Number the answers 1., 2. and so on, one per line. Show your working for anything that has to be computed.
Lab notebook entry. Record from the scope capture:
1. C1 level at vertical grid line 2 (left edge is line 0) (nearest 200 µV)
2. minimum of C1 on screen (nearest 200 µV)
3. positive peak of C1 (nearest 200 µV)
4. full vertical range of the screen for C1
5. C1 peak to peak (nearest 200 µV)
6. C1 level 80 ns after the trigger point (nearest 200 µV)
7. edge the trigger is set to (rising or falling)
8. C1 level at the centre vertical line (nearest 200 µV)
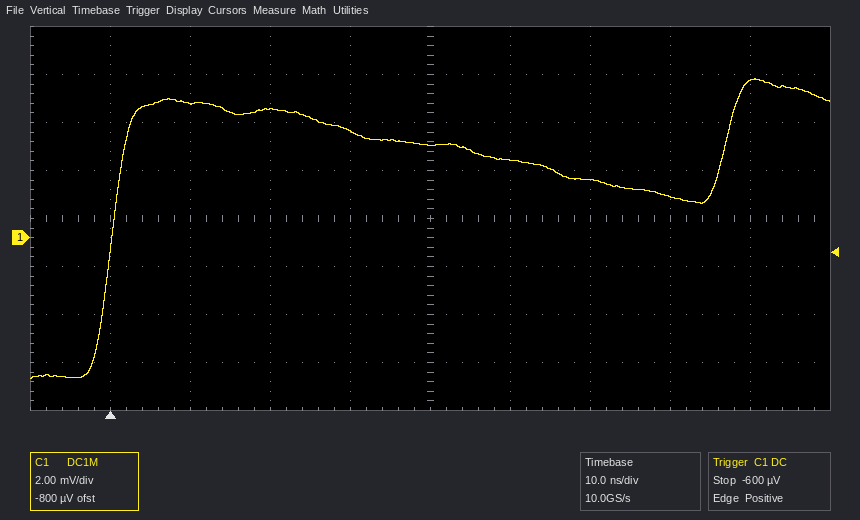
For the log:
1. 5.6 mV
2. -5.8 mV
3. 6.6 mV
4. 16 mV
5. 6.6 mV − (-5.8 mV) = 12.4 mV
6. 6.6 mV
7. rising
8. 3.8 mV
